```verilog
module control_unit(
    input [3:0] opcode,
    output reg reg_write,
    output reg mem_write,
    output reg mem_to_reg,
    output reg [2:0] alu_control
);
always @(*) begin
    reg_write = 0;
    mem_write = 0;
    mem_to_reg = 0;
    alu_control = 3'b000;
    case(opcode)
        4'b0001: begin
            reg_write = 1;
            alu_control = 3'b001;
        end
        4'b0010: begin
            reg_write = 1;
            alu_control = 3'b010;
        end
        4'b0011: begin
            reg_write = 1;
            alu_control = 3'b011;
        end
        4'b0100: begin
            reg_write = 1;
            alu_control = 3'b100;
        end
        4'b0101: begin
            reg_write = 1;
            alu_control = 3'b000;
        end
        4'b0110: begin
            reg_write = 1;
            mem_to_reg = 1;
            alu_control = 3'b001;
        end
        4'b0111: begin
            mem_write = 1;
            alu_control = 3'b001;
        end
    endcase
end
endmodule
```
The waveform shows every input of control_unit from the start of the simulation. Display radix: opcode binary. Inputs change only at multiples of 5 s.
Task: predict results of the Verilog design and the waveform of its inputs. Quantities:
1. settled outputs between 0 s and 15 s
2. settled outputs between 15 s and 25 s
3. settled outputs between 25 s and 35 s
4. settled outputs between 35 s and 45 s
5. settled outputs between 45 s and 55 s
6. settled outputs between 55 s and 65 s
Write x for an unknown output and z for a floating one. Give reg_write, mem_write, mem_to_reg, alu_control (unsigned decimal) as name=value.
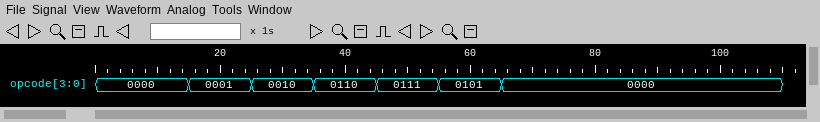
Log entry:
reg_write=0, mem_write=0, mem_to_reg=0, alu_control=0
reg_write=1, mem_write=0, mem_to_reg=0, alu_control=1
reg_write=1, mem_write=0, mem_to_reg=0, alu_control=2
reg_write=1, mem_write=0, mem_to_reg=1, alu_control=1
reg_write=0, mem_write=1, mem_to_reg=0, alu_control=1
reg_write=1, mem_write=0, mem_to_reg=0, alu_control=0
